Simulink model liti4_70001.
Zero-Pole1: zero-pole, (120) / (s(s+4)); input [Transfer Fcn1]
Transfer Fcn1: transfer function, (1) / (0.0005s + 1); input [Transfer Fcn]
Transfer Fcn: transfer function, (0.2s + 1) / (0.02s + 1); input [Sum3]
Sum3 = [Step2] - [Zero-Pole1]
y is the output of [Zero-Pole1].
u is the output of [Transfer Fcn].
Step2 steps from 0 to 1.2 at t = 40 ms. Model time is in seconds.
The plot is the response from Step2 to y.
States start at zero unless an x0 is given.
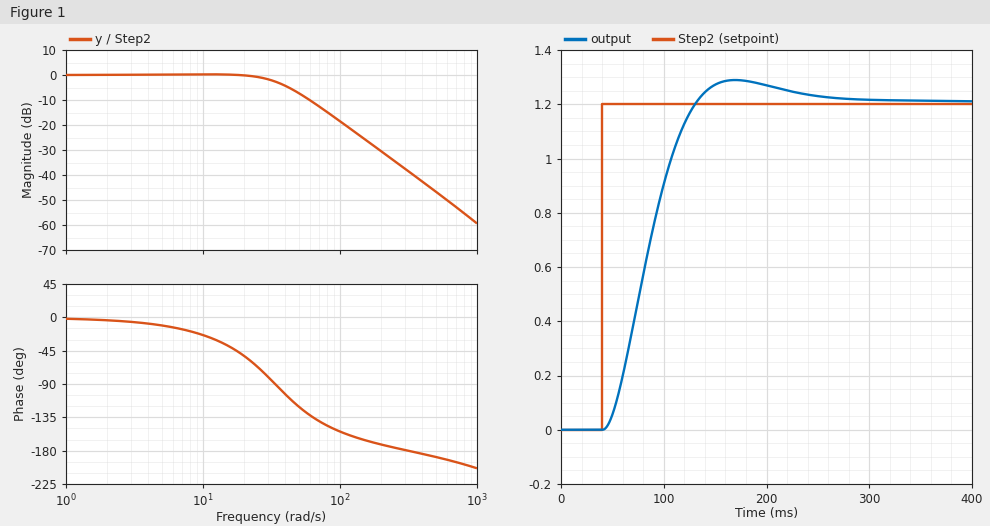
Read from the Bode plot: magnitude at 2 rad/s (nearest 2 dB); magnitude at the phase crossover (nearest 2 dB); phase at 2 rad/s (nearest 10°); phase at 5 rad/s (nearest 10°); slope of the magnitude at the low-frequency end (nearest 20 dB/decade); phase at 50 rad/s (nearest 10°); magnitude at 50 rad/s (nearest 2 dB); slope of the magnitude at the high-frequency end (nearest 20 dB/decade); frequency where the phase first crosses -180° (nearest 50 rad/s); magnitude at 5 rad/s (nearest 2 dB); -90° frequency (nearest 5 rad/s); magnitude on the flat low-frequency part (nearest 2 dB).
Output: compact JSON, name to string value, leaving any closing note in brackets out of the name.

{"magnitude at 2 rad/s": "0 dB", "magnitude at the phase crossover": "-38 dB", "phase at 2 rad/s": "0°", "phase at 5 rad/s": "-10°", "slope of the magnitude at the low-frequency end": "0 dB/decade", "phase at 50 rad/s": "-120°", "magnitude at 50 rad/s": "-8 dB", "slope of the magnitude at the high-frequency end": "-40 dB/decade", "frequency where the phase first crosses -180°": "300 rad/s", "magnitude at 5 rad/s": "0 dB", "-90° frequency": "35 rad/s", "magnitude on the flat low-frequency part": "0 dB"}
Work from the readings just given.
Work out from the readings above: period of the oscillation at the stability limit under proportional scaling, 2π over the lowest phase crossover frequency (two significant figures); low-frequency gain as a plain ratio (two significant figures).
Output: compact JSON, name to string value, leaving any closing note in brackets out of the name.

{"period of the oscillation at the stability limit under proportional scaling, 2π over the lowest phase crossover frequency": "0.021 s", "low-frequency gain as a plain ratio": "1.0"}
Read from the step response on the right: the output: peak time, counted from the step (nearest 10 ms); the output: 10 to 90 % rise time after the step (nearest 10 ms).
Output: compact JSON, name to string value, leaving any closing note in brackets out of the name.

{"the output: peak time, counted from the step": "130 ms", "the output: 10 to 90 % rise time after the step": "60 ms"}
